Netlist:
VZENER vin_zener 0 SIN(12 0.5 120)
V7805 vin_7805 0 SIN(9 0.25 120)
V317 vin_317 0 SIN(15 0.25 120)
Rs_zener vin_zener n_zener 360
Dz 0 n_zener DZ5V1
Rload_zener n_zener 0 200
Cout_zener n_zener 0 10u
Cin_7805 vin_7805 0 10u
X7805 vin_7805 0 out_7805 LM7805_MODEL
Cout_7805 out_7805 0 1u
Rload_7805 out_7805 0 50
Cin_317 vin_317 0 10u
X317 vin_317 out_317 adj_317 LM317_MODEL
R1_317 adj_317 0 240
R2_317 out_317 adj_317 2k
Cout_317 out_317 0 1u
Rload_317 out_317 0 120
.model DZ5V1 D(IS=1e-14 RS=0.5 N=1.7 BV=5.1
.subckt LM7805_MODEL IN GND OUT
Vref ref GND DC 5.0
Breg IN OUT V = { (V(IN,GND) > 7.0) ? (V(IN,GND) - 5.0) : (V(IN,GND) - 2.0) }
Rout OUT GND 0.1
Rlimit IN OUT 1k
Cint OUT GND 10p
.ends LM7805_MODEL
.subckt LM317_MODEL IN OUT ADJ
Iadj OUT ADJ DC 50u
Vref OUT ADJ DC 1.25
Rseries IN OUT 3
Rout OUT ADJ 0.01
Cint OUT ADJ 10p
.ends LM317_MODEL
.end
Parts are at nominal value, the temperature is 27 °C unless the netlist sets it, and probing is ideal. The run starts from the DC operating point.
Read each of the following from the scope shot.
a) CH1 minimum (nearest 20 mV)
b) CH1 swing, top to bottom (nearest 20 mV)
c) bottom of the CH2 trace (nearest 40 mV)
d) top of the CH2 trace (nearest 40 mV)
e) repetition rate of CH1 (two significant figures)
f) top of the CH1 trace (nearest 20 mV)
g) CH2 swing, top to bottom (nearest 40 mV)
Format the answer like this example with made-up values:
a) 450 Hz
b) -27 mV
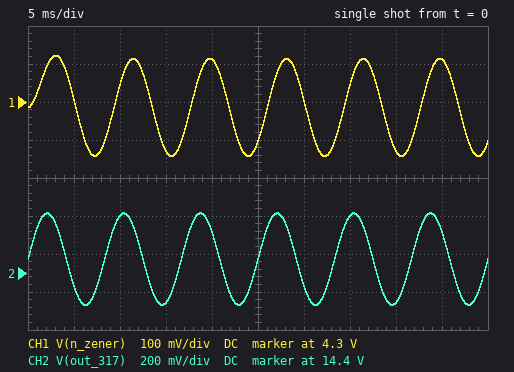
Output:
a) 4.16 V
b) 260 mV
c) 14.24 V
d) 14.72 V
e) 120 Hz
f) 4.42 V
g) 480 mV
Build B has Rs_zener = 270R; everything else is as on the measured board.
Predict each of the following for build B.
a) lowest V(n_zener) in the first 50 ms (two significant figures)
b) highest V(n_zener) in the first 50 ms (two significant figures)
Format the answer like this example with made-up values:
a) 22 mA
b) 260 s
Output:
a) 4.9 V
b) 5.1 V
